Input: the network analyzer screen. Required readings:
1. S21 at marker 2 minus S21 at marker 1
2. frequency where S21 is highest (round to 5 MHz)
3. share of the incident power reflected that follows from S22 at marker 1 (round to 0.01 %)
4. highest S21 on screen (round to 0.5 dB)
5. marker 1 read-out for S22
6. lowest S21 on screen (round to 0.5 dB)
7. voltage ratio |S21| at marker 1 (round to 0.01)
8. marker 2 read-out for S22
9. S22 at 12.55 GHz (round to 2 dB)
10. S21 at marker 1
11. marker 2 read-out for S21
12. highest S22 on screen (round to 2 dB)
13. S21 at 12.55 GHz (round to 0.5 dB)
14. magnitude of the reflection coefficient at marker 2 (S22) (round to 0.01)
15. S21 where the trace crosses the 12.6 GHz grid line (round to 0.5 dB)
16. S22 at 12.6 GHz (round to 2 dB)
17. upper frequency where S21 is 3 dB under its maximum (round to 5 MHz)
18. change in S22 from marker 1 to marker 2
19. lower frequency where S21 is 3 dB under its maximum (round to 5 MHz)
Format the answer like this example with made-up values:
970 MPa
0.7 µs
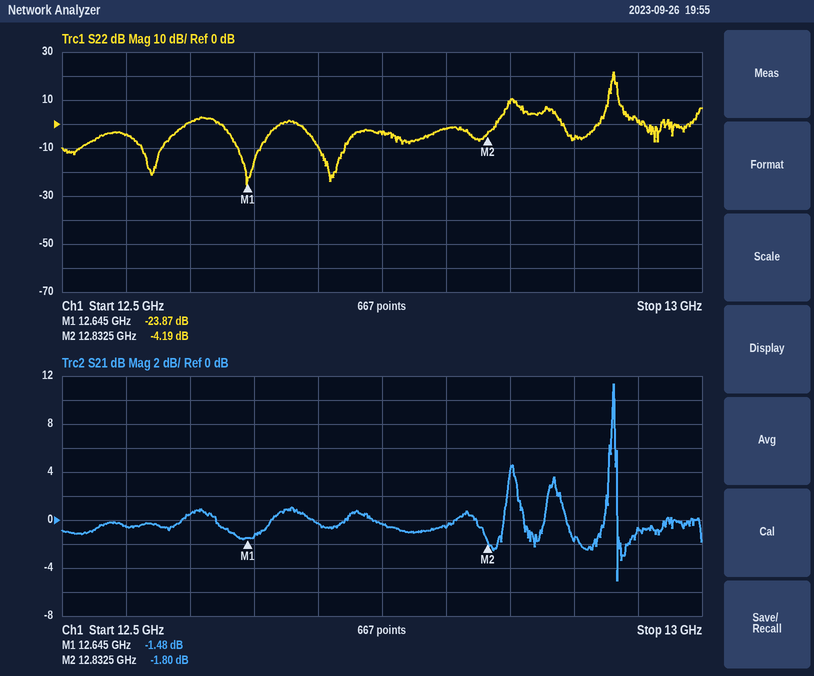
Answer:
-0.32 dB
12.930 GHz
0.41 %
11.5 dB
-23.87 dB
-5.0 dB
0.84
-4.19 dB
-4 dB
-1.48 dB
-1.80 dB
22 dB
-0.5 dB
0.62
0.5 dB
0 dB
12.930 GHz
19.68 dB
12.930 GHz
